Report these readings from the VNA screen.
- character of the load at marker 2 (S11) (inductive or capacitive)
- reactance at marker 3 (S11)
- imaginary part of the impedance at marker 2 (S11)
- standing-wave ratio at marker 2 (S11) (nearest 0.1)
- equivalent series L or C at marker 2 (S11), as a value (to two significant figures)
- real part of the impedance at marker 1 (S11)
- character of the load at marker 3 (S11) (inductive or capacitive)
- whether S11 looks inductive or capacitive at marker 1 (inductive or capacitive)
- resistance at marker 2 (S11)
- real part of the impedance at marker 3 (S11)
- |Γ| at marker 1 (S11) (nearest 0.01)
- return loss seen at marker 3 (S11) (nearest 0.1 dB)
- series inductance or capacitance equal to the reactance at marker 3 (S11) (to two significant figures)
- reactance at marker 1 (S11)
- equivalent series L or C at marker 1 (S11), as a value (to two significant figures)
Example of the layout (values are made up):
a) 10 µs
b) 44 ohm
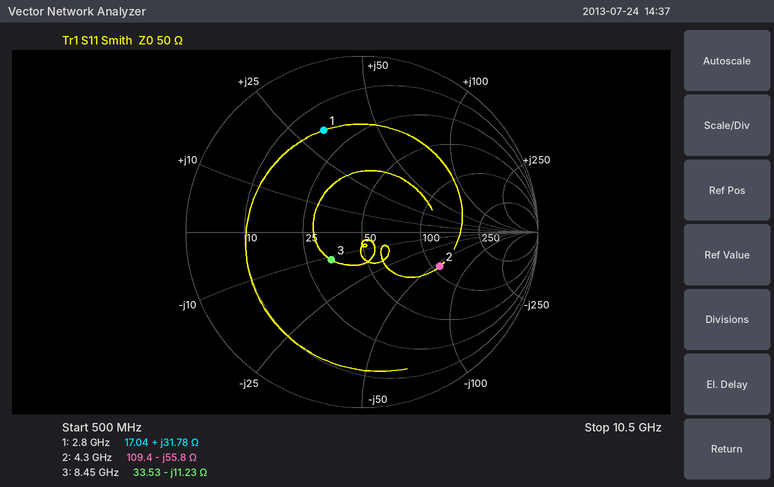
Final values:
a) capacitive
b) -11.23 Ω
c) -55.8 Ω
d) 2.9
e) 660 fF
f) 17.04 Ω
g) capacitive
h) inductive
i) 109.4 Ω
j) 33.53 Ω
k) 0.62
l) 12.5 dB
m) 1.7 pF
n) +31.78 Ω
o) 1.8 nH
